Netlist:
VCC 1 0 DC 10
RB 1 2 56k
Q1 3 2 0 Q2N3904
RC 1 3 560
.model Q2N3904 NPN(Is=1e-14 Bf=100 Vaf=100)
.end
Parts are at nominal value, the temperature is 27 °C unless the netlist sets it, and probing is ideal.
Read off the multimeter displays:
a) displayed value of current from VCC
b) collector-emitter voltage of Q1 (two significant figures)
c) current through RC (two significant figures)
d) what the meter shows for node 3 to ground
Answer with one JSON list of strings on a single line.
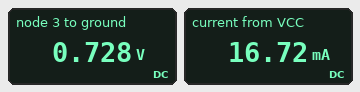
["16.72 mA", "730 mV", "17 mA", "0.728 V"]
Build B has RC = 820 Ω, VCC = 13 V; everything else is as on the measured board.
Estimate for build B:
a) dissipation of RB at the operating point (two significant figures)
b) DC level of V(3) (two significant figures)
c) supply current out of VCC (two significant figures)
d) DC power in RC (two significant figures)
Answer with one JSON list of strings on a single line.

["2.7 mW", "140 mV", "16 mA", "200 mW"]
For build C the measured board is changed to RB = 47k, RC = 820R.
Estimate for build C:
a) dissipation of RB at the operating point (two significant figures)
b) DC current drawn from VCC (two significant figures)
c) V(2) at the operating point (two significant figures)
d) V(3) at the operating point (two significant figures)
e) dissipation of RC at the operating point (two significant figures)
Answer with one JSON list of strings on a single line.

["1.8 mW", "12 mA", "720 mV", "130 mV", "120 mW"]
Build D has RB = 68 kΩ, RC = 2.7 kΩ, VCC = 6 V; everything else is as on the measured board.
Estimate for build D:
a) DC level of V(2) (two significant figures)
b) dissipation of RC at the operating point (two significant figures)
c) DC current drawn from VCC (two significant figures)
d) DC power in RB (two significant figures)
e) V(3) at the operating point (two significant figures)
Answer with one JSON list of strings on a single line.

["680 mV", "13 mW", "2.3 mA", "420 µW", "97 mV"]
